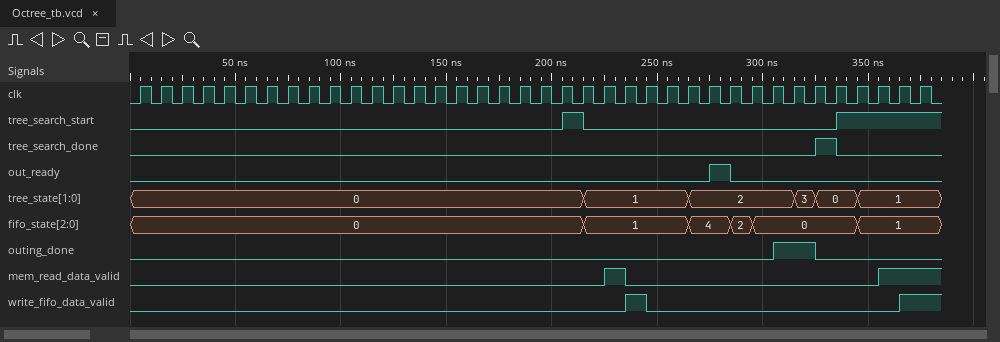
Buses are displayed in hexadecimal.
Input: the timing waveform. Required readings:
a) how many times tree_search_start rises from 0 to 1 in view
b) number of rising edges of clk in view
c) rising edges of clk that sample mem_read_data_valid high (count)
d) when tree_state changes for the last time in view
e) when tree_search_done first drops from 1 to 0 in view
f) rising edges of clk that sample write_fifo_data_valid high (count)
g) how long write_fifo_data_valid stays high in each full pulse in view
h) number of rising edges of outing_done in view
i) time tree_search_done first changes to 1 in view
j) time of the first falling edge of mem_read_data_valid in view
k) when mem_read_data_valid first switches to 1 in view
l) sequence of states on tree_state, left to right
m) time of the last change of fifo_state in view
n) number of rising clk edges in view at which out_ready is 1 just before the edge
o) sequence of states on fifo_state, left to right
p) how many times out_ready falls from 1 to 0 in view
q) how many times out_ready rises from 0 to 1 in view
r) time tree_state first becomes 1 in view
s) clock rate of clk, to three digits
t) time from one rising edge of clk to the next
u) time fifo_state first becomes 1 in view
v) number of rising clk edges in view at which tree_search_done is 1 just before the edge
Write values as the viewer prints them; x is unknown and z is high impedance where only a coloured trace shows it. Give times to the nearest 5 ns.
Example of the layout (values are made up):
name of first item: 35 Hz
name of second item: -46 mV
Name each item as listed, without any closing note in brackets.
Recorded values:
how many times tree_search_start rises from 0 to 1 in view: 2
number of rising edges of clk in view: 38
rising edges of clk that sample mem_read_data_valid high: 3
when tree_state changes for the last time in view: 345 ns
when tree_search_done first drops from 1 to 0 in view: 335 ns
rising edges of clk that sample write_fifo_data_valid high: 2
how long write_fifo_data_valid stays high in each full pulse in view: 10 ns
number of rising edges of outing_done in view: 1
time tree_search_done first changes to 1 in view: 325 ns
time of the first falling edge of mem_read_data_valid in view: 235 ns
when mem_read_data_valid first switches to 1 in view: 225 ns
sequence of states on tree_state, left to right: 0, 1, 2, 3, 0, 1
time of the last change of fifo_state in view: 345 ns
number of rising clk edges in view at which out_ready is 1 just before the edge: 1
sequence of states on fifo_state, left to right: 0, 1, 4, 2, 0, 1
how many times out_ready falls from 1 to 0 in view: 1
how many times out_ready rises from 0 to 1 in view: 1
time tree_state first becomes 1 in view: 215 ns
clock rate of clk, to three digits: 100 MHz
time from one rising edge of clk to the next: 10 ns
time fifo_state first becomes 1 in view: 215 ns
number of rising clk edges in view at which tree_search_done is 1 just before the edge: 1
